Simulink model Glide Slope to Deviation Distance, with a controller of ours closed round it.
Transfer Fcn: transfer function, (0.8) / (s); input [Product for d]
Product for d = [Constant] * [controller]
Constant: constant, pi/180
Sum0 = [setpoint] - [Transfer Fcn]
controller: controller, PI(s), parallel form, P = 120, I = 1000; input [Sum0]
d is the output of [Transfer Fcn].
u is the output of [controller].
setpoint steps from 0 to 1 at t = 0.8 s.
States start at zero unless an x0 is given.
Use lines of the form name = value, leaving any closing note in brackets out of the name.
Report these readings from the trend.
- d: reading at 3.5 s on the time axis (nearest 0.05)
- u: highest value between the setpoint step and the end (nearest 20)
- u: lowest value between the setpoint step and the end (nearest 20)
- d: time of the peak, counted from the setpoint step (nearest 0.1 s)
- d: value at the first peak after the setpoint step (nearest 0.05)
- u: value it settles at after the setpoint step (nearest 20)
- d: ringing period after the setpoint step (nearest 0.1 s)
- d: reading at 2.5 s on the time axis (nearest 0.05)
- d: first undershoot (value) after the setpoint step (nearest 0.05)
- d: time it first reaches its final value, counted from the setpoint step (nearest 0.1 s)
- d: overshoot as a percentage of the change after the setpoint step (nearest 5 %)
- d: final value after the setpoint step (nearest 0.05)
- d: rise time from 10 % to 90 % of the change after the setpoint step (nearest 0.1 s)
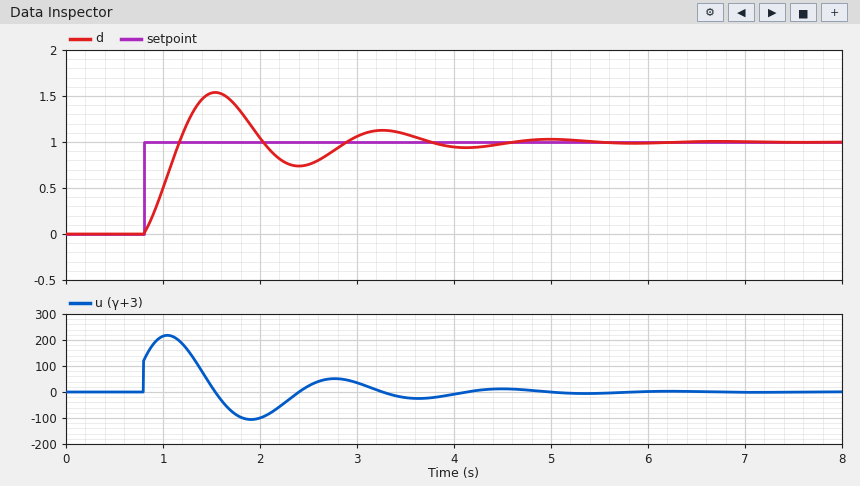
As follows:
d: reading at 3.5 s on the time axis = 1.10
u: highest value between the setpoint step and the end = 220
u: lowest value between the setpoint step and the end = -100
d: time of the peak, counted from the setpoint step = 0.7 s
d: value at the first peak after the setpoint step = 1.55
u: value it settles at after the setpoint step = 0
d: ringing period after the setpoint step = 1.7 s
d: reading at 2.5 s on the time axis = 0.75
d: first undershoot (value) after the setpoint step = 0.75
d: time it first reaches its final value, counted from the setpoint step = 0.4 s
d: overshoot as a percentage of the change after the setpoint step = 55 %
d: final value after the setpoint step = 1.00
d: rise time from 10 % to 90 % of the change after the setpoint step = 0.3 s
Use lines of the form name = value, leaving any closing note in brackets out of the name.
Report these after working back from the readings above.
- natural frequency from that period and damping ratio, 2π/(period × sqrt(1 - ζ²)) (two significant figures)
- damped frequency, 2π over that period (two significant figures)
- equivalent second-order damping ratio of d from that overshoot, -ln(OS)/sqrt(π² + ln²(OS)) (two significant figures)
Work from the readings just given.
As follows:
natural frequency from that period and damping ratio, 2π/(period × sqrt(1 - ζ²)) = 3.8 rad/s
damped frequency, 2π over that period = 3.7 rad/s
equivalent second-order damping ratio of d from that overshoot, -ln(OS)/sqrt(π² + ln²(OS)) = 0.19
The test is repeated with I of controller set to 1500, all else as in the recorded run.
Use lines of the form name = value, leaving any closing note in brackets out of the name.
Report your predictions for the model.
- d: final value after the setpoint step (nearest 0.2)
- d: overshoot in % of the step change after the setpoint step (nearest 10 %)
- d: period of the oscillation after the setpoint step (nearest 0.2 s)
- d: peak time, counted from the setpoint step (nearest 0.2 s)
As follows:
d: final value after the setpoint step = 1.0
d: overshoot in % of the step change after the setpoint step = 60 %
d: period of the oscillation after the setpoint step = 1.4 s
d: peak time, counted from the setpoint step = 0.6 s
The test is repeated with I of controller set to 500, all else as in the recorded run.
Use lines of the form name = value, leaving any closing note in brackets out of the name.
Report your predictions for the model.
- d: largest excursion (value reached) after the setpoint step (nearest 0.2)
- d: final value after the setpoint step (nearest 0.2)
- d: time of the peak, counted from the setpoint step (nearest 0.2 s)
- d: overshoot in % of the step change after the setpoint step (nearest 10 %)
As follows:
d: largest excursion (value reached) after the setpoint step = 1.4
d: final value after the setpoint step = 1.0
d: time of the peak, counted from the setpoint step = 1.0 s
d: overshoot in % of the step change after the setpoint step = 40 %
